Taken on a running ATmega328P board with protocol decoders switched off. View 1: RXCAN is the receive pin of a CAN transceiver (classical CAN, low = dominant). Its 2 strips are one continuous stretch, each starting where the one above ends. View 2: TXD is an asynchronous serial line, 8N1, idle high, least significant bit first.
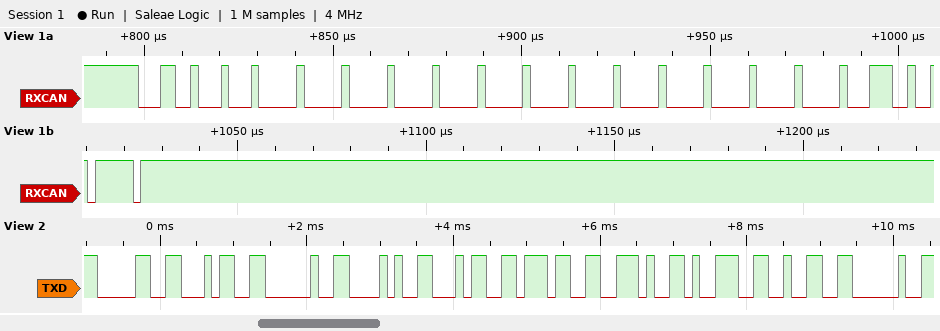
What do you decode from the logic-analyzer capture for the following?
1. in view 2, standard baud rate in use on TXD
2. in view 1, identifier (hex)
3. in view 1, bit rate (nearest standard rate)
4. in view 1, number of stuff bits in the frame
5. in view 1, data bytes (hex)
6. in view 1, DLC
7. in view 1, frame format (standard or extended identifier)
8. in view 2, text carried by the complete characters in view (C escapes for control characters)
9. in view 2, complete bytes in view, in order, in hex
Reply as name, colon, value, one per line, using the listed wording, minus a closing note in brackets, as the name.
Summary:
in view 2, standard baud rate in use on TXD: 9600 baud
in view 1, identifier: 0x191
in view 1, bit rate: 500 kbit/s
in view 1, number of stuff bits in the frame: 13
in view 1, data bytes: 00 00 00 00 00 00 00 00
in view 1, DLC: 8
in view 1, frame format: standard
in view 2, text carried by the complete characters in view: "04 (47.92 "
in view 2, complete bytes in view, in order, in hex: 0x30 0x34 0x20 0x28 0x34 0x37 0x2E 0x39 0x32 0x20
